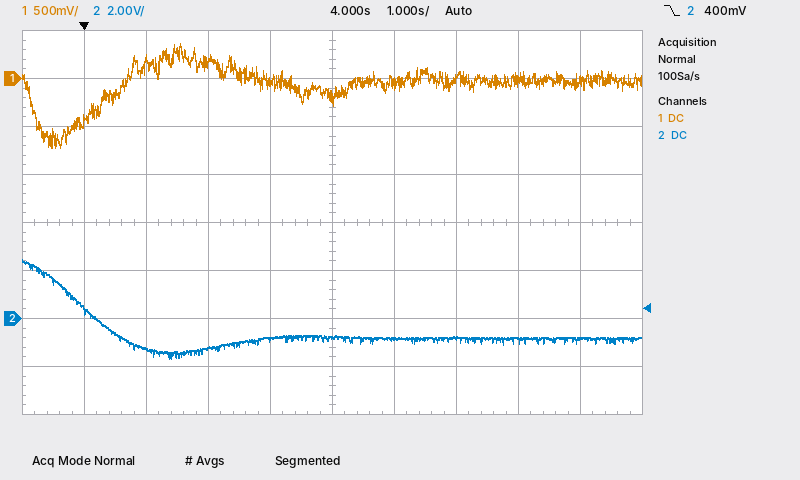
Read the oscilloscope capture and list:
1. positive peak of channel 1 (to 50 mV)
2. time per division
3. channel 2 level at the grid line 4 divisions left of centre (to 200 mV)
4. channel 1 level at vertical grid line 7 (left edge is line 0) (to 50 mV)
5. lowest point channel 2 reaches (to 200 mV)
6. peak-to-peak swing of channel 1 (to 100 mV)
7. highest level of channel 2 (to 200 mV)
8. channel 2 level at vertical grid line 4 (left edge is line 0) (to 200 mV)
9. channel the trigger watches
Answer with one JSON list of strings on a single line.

["350 mV", "1 s", "400 mV", "0 mV", "-1.6 V", "1.10 V", "2.4 V", "-800 mV", "channel 2"]
